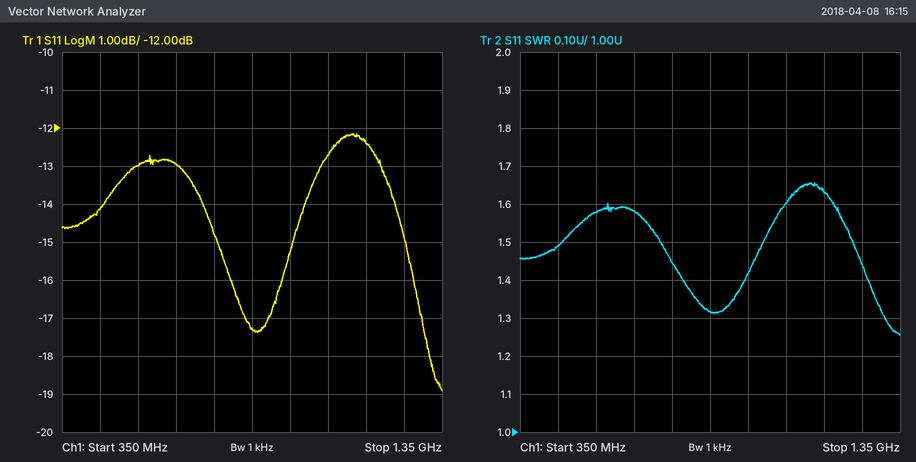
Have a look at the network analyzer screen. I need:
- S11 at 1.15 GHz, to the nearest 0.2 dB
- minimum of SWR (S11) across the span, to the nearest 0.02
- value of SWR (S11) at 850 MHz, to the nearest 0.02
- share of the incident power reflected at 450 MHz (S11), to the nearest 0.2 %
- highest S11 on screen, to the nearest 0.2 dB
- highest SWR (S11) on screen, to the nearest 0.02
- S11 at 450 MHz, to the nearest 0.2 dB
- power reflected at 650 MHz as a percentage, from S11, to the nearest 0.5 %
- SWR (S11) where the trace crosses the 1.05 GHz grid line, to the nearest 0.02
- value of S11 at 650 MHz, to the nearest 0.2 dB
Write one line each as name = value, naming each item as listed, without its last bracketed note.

S11 at 1.15 GHz, to the nearest 0.2 dB = -12.4 dB
minimum of SWR (S11) across the span, to the nearest 0.02 = 1.26
value of SWR (S11) at 850 MHz, to the nearest 0.02 = 1.32
share of the incident power reflected at 450 MHz (S11), to the nearest 0.2 % = 3.8 %
highest S11 on screen, to the nearest 0.2 dB = -12.2 dB
highest SWR (S11) on screen, to the nearest 0.02 = 1.66
S11 at 450 MHz, to the nearest 0.2 dB = -14.2 dB
power reflected at 650 MHz as a percentage, from S11, to the nearest 0.5 % = 5.0 %
SWR (S11) where the trace crosses the 1.05 GHz grid line, to the nearest 0.02 = 1.60
value of S11 at 650 MHz, to the nearest 0.2 dB = -13.0 dB
